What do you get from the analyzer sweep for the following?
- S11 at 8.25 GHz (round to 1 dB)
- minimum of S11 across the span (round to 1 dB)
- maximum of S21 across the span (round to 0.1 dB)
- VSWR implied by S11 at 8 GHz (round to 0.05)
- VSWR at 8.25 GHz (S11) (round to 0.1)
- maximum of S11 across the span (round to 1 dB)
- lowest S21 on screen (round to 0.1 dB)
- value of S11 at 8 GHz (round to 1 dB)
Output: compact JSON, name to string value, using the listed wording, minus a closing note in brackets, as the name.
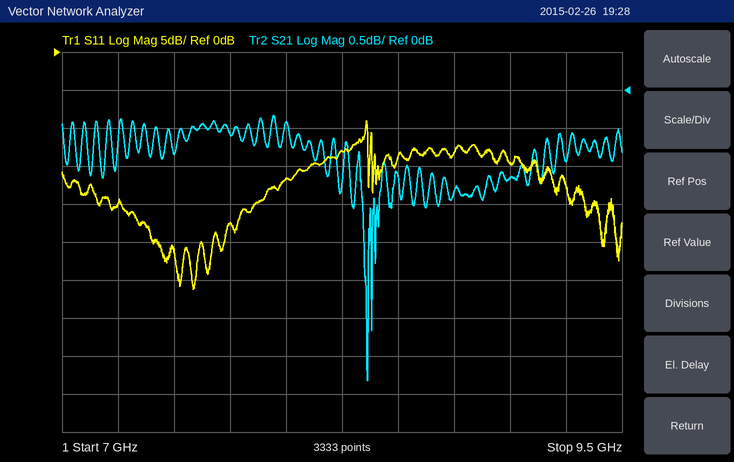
{"S11 at 8.25 GHz": "-13 dB", "minimum of S11 across the span": "-31 dB", "maximum of S21 across the span": "-0.3 dB", "VSWR implied by S11 at 8 GHz": "1.35", "VSWR at 8.25 GHz (S11)": "1.6", "maximum of S11 across the span": "-9 dB", "lowest S21 on screen": "-3.8 dB", "value of S11 at 8 GHz": "-17 dB"}
